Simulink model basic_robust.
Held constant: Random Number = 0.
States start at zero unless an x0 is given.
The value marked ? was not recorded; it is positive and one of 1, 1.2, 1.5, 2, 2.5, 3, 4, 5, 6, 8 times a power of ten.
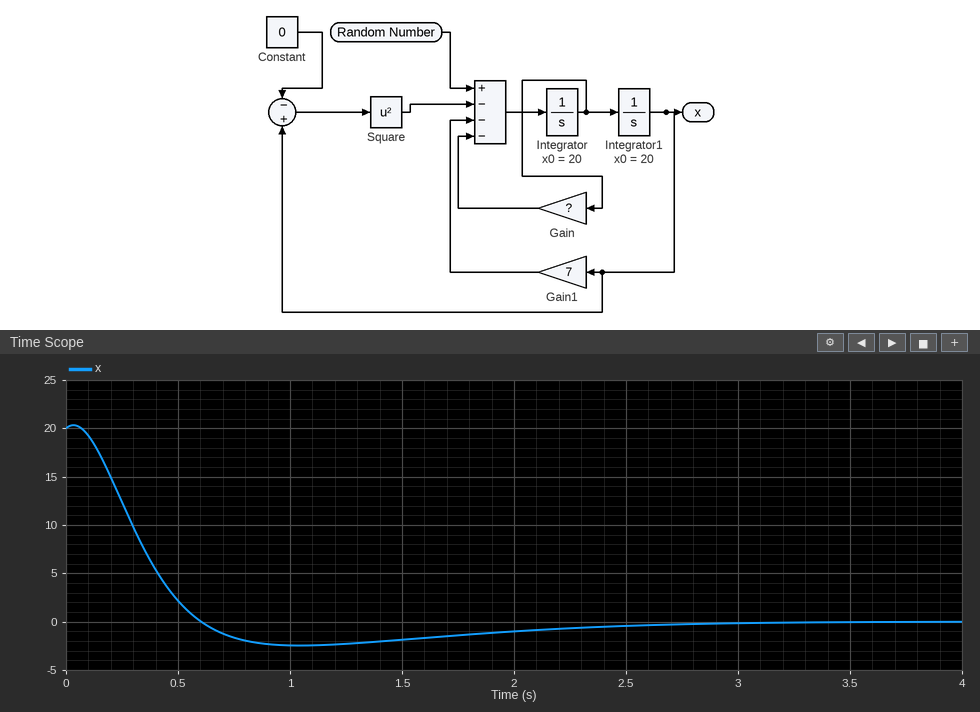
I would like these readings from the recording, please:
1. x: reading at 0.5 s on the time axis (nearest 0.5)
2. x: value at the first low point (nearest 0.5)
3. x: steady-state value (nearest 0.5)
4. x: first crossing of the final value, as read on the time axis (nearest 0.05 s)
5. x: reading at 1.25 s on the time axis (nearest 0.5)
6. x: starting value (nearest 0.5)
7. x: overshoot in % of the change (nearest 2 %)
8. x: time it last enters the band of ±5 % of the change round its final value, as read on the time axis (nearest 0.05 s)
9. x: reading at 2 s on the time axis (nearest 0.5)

2.0
-2.5
0.0
0.60 s
-2.5
20.0
12 %
2.00 s
-1.0
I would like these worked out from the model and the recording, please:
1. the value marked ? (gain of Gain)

5
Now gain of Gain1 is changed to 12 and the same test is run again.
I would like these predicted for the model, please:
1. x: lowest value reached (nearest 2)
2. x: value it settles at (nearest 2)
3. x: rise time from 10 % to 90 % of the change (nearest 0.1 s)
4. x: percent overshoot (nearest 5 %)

-4
0
0.3 s
20 %
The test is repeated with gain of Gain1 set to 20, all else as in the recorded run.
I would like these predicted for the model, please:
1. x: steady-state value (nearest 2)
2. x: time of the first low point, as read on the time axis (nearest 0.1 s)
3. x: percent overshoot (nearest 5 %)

0
0.7 s
25 %
